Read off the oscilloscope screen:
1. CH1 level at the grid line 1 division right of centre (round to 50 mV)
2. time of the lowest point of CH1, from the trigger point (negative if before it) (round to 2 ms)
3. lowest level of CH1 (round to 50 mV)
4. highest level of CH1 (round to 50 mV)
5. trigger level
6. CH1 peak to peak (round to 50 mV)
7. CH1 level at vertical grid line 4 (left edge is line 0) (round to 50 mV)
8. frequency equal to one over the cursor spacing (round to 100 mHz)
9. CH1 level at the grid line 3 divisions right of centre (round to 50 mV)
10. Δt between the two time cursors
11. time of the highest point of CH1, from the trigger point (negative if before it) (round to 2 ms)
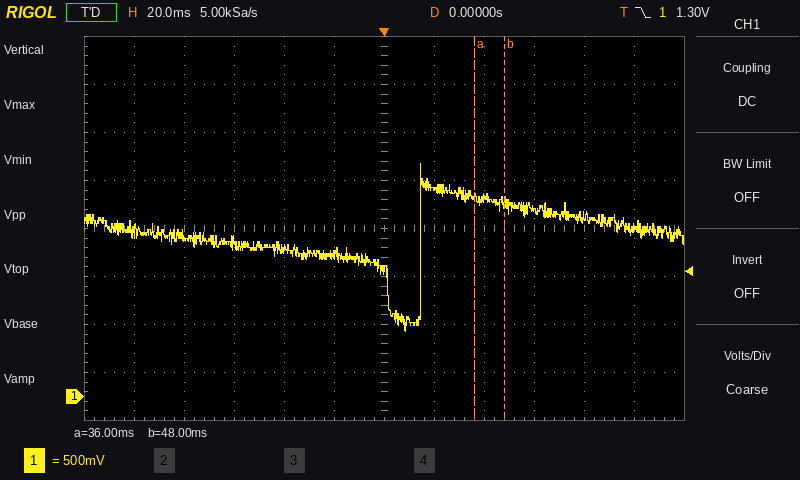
2.15 V
+8 ms
700 mV
2.45 V
1.30 V
1.75 V
1.55 V
83.3 Hz
1.95 V
12 ms
+14 ms
